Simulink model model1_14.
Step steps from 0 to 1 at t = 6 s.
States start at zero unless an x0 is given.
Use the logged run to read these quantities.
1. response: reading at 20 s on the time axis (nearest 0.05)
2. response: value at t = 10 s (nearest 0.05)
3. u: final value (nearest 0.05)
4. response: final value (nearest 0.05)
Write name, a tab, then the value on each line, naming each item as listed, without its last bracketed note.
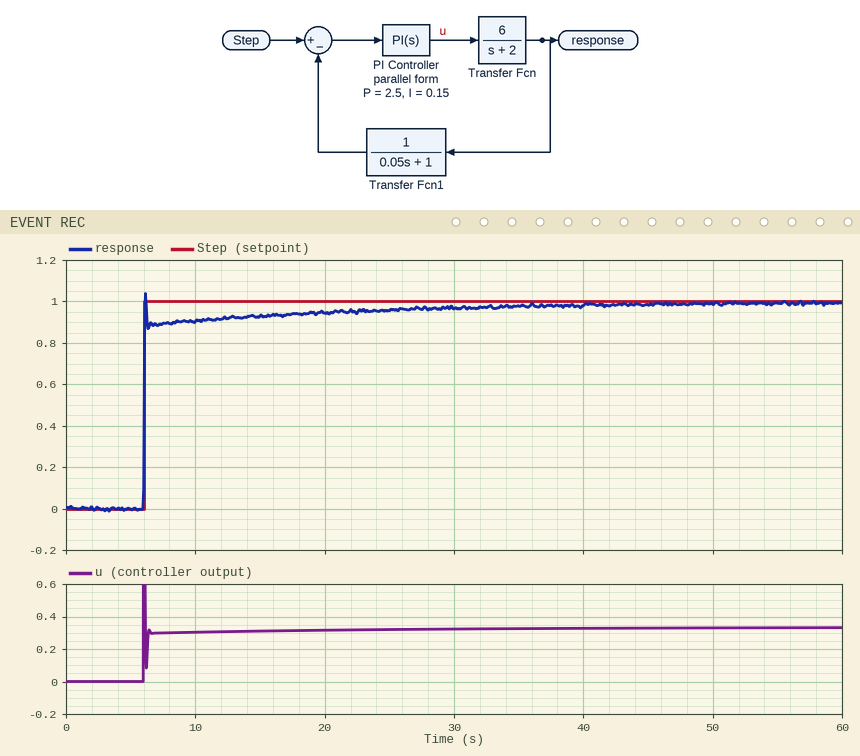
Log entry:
response: reading at 20 s on the time axis	0.95
response: value at t = 10 s	0.90
u: final value	0.35
response: final value	1.00
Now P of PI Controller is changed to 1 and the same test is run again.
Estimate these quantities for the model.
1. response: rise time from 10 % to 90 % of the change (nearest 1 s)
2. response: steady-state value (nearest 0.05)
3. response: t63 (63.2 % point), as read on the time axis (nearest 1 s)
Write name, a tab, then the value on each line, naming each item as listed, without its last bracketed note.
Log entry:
response: rise time from 10 % to 90 % of the change	8 s
response: steady-state value	1.00
response: t63 (63.2 % point), as read on the time axis	6 s
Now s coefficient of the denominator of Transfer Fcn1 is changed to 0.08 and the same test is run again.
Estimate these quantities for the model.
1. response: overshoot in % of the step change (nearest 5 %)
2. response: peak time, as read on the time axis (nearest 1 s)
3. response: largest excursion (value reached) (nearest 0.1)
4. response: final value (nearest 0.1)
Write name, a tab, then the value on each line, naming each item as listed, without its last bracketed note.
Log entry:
response: overshoot in % of the step change	20 %
response: peak time, as read on the time axis	6 s
response: largest excursion (value reached)	1.2
response: final value	1.0
